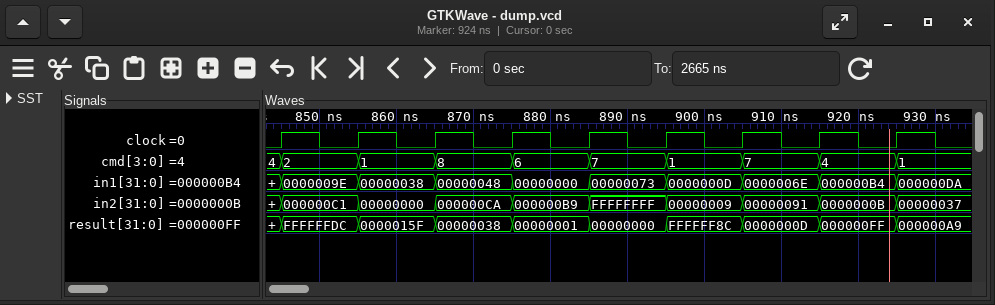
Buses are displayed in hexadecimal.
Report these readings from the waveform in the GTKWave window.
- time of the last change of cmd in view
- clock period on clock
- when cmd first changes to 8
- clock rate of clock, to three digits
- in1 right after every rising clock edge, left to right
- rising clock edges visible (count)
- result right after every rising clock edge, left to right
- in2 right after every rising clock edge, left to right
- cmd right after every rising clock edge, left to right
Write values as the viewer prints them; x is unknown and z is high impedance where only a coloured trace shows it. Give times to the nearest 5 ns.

925 ns
10 ns
865 ns
100 MHz
0000009E, 00000038, 00000048, 00000000, 00000073, 0000000D, 0000006E, 000000B4, 000000DA
9
FFFFFFDC, 0000015F, 00000038, 00000001, 00000000, FFFFFF8C, 0000000D, 000000FF, 000000A9
000000C1, 00000000, 000000CA, 000000B9, FFFFFFFF, 00000009, 00000091, 0000000B, 00000037
2, 1, 8, 6, 7, 1, 7, 4, 1
